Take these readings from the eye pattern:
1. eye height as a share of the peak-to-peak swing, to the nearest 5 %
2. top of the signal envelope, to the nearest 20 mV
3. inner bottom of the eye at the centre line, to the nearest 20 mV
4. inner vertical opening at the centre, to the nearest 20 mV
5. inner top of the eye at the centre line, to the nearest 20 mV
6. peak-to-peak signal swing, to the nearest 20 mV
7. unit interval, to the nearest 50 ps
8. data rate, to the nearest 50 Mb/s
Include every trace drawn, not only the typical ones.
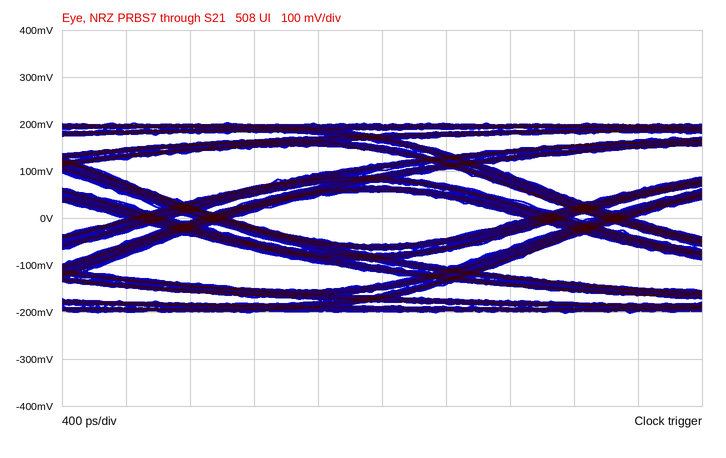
30 %
200 mV
-60 mV
120 mV
60 mV
400 mV
2.50 ns
400 Mb/s
